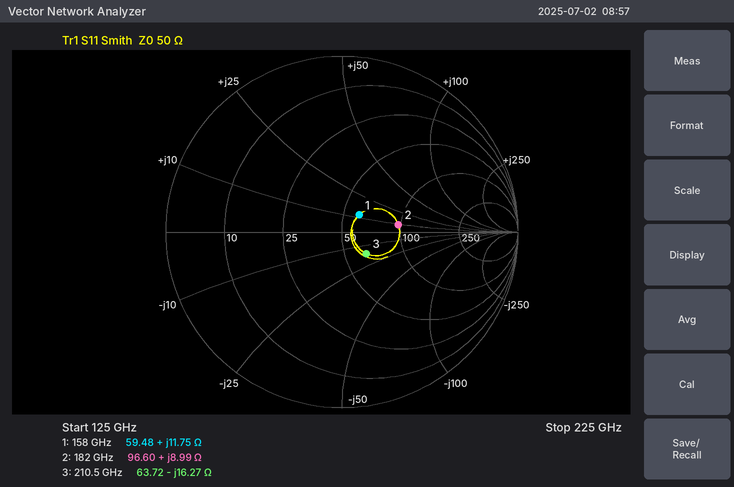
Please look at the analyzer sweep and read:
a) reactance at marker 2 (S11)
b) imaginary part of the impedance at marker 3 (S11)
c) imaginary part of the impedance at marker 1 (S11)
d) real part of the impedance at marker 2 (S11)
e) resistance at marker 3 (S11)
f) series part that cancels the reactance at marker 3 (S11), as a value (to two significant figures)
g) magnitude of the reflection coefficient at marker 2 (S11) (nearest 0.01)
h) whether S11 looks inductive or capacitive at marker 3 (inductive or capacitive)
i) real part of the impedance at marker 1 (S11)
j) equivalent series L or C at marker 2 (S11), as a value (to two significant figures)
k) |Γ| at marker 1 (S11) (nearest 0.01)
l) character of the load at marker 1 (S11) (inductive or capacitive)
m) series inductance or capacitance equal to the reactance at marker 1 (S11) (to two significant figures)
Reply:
+8.99 Ω
-16.27 Ω
+11.75 Ω
96.60 Ω
63.72 Ω
12 pH
0.32
capacitive
59.48 Ω
7.9 pH
0.14
inductive
12 pH
